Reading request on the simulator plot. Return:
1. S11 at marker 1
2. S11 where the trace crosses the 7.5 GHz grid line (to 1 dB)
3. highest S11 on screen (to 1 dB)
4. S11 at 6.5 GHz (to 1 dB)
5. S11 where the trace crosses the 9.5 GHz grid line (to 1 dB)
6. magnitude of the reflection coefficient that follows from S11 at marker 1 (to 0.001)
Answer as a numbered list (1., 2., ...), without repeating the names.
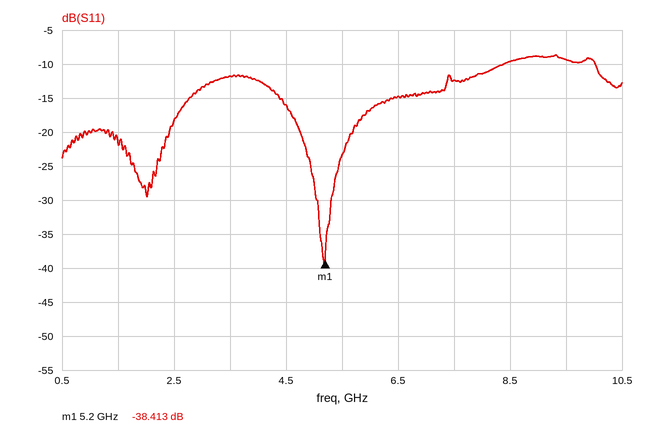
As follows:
1. -38.413 dB
2. -12 dB
3. -9 dB
4. -15 dB
5. -9 dB
6. 0.012
